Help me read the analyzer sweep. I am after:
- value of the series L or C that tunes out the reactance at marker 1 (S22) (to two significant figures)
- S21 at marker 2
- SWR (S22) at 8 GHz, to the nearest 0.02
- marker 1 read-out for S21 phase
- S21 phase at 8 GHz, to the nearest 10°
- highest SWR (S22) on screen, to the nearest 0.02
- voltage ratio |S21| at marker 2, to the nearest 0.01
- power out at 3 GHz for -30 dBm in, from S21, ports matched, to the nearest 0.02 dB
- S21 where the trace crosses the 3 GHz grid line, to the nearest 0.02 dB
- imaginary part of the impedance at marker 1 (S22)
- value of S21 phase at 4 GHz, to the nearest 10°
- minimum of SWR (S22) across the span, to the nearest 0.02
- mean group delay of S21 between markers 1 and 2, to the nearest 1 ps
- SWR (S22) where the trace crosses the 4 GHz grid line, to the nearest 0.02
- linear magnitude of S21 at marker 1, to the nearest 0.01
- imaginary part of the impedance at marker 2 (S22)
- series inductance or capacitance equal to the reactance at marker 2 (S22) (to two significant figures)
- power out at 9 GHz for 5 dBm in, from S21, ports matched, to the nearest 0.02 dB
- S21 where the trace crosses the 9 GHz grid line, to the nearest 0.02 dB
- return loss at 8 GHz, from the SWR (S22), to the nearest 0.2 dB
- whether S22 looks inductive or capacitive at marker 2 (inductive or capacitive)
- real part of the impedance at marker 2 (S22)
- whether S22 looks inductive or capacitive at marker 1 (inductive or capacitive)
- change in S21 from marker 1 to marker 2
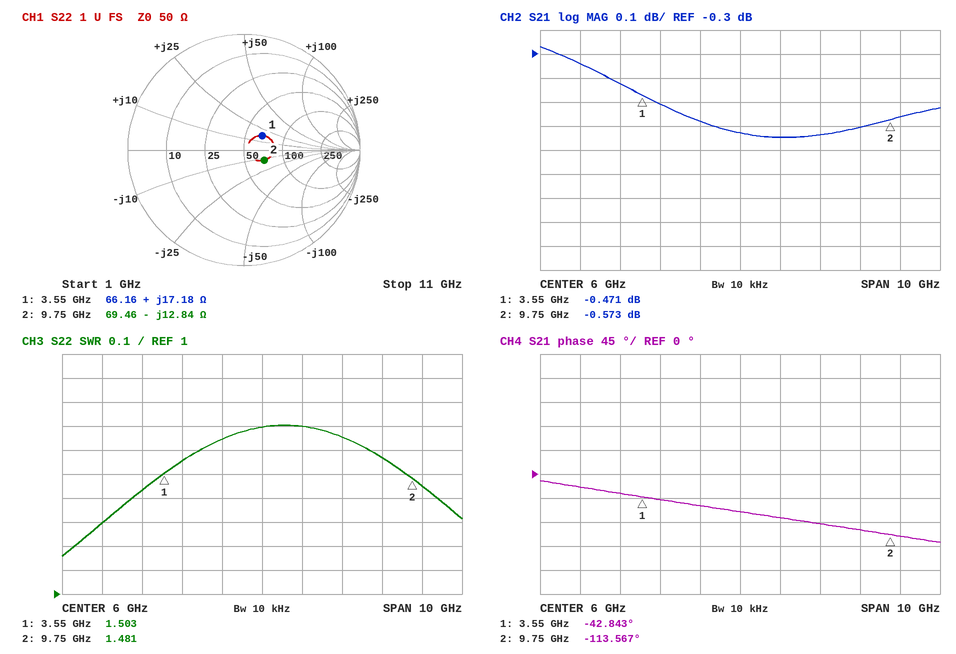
2.6 pF
-0.573 dB
1.66
-42.843°
-90°
1.70
0.94
-30.42 dBm
-0.42 dB
+17.18 Ω
-50°
1.16
32 ps
1.56
0.95
-12.84 Ω
1.3 pF
4.40 dBm
-0.60 dB
12.2 dB
capacitive
69.46 Ω
inductive
-0.102 dB
